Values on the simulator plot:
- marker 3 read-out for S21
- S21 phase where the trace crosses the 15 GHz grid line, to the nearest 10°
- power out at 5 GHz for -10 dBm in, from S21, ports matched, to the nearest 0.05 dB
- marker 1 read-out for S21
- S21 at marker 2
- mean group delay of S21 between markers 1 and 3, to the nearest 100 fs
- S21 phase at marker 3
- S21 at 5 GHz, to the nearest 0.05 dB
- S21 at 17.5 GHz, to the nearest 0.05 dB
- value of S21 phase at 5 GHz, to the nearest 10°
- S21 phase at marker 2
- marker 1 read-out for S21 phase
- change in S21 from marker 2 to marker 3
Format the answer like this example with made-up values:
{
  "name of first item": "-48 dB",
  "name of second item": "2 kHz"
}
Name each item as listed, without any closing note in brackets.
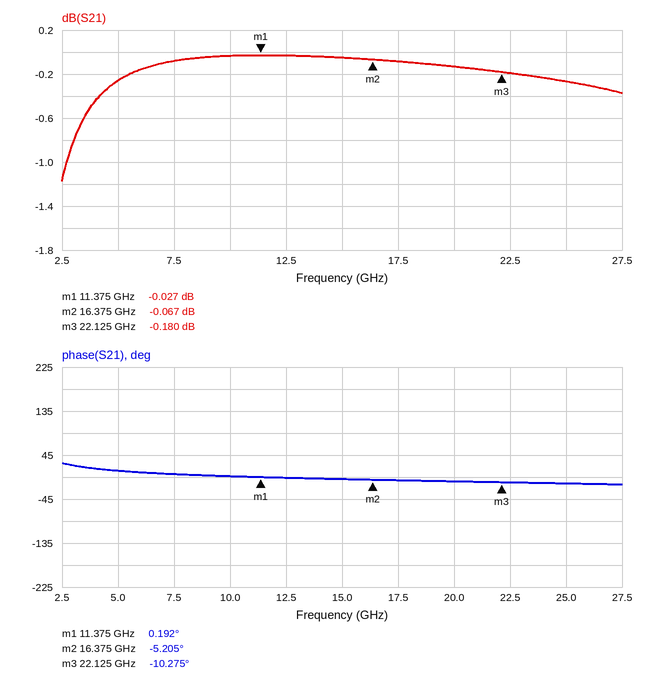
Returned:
{
  "marker 3 read-out for S21": "-0.180 dB",
  "S21 phase where the trace crosses the 15 GHz grid line, to the nearest 10°": "0°",
  "power out at 5 GHz for -10 dBm in, from S21, ports matched, to the nearest 0.05 dB": "-10.25 dBm",
  "marker 1 read-out for S21": "-0.027 dB",
  "S21 at marker 2": "-0.067 dB",
  "mean group delay of S21 between markers 1 and 3, to the nearest 100 fs": "2.7 ps",
  "S21 phase at marker 3": "-10.275°",
  "S21 at 5 GHz, to the nearest 0.05 dB": "-0.25 dB",
  "S21 at 17.5 GHz, to the nearest 0.05 dB": "-0.10 dB",
  "value of S21 phase at 5 GHz, to the nearest 10°": "10°",
  "S21 phase at marker 2": "-5.205°",
  "marker 1 read-out for S21 phase": "0.192°",
  "change in S21 from marker 2 to marker 3": "-0.113 dB"
}
